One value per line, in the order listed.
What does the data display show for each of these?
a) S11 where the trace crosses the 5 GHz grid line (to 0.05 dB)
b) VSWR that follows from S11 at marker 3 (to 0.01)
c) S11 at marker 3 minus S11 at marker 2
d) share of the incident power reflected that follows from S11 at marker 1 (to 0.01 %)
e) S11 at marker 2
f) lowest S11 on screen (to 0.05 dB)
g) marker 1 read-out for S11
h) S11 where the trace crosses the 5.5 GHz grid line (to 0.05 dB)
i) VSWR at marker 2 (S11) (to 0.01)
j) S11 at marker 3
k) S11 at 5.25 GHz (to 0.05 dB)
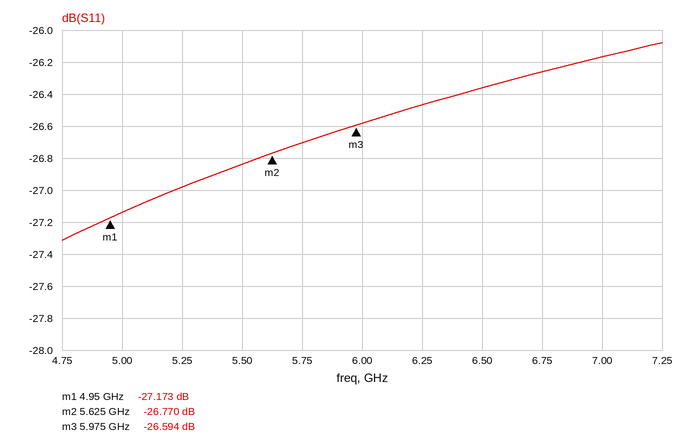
-27.15 dB
1.10
0.176 dB
0.19 %
-26.770 dB
-27.30 dB
-27.173 dB
-26.85 dB
1.10
-26.594 dB
-27.00 dB
